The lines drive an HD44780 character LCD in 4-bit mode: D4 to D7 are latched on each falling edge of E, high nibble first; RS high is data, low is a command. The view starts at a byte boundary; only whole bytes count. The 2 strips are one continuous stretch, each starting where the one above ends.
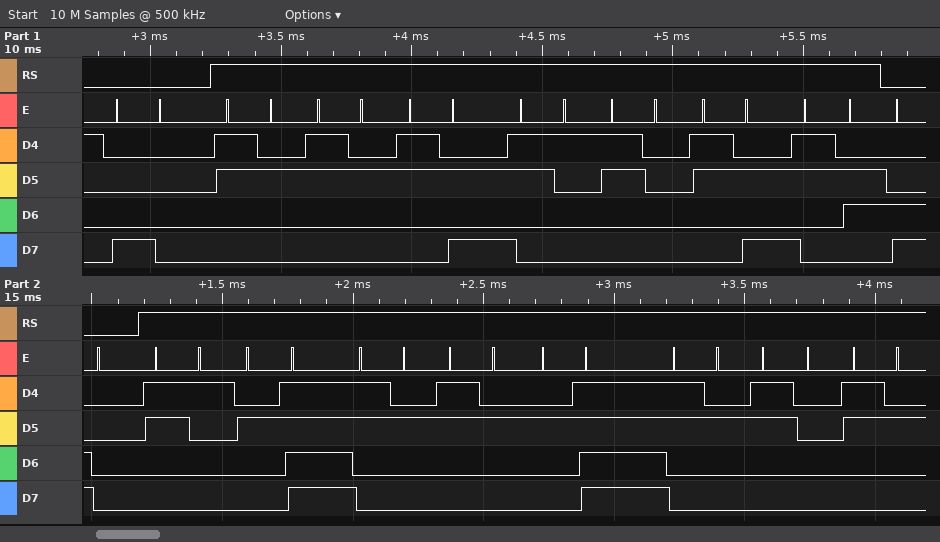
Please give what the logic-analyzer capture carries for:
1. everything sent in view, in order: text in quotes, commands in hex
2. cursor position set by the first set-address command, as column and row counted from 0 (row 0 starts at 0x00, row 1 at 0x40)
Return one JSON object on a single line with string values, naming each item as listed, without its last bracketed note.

{"everything sent in view, in order: text in quotes, commands in hex": "0x80 \"22:10:6\" 0xC0 \"1/22/202\"", "cursor position set by the first set-address command, as column and row counted from 0": "column 0, row 0"}
